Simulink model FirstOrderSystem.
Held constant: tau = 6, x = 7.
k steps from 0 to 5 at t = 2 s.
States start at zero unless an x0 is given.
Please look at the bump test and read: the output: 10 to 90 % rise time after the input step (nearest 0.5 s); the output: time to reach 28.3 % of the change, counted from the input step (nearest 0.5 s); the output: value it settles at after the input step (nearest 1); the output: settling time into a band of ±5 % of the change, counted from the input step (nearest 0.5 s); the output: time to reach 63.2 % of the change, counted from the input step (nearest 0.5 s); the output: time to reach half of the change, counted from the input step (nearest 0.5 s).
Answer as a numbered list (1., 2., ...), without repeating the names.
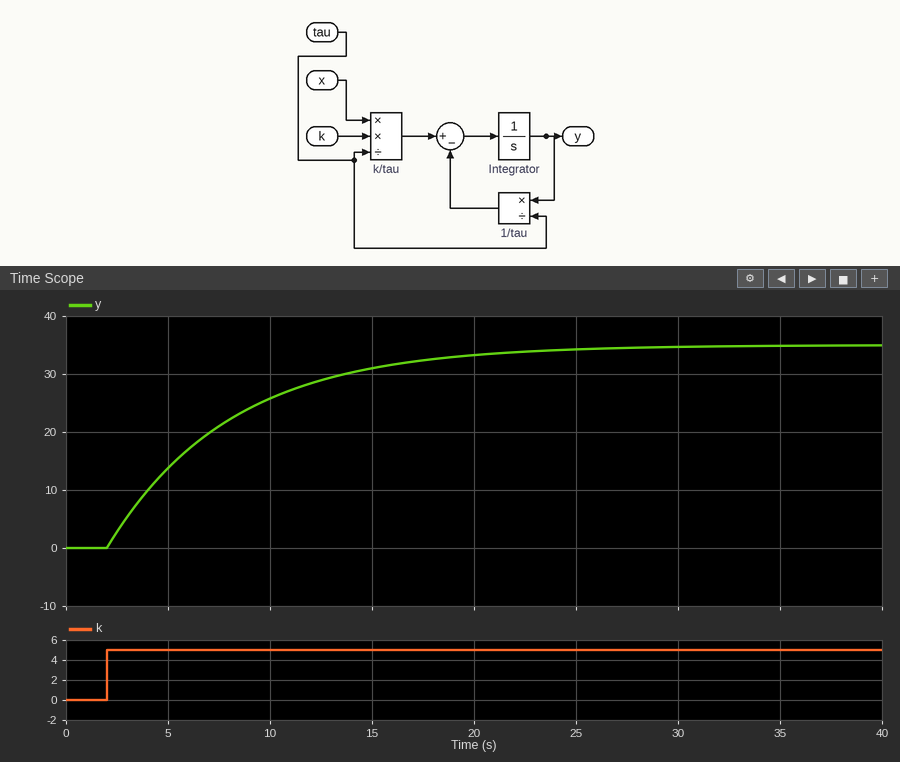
1. 13.0 s
2. 2.0 s
3. 35
4. 18.0 s
5. 6.0 s
6. 4.0 s
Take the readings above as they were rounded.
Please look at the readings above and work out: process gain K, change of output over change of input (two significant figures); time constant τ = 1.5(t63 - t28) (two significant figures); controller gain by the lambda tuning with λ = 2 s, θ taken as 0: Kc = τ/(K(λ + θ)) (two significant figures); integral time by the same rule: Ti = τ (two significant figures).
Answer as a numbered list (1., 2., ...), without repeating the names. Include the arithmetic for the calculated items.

1. (35 - 0) / 5 = 7.0
2. 1.5 × (6 - 2) = 6.0 s
3. 6 / (7 × (2 + 0)) = 0.43
4. 6.0 s
